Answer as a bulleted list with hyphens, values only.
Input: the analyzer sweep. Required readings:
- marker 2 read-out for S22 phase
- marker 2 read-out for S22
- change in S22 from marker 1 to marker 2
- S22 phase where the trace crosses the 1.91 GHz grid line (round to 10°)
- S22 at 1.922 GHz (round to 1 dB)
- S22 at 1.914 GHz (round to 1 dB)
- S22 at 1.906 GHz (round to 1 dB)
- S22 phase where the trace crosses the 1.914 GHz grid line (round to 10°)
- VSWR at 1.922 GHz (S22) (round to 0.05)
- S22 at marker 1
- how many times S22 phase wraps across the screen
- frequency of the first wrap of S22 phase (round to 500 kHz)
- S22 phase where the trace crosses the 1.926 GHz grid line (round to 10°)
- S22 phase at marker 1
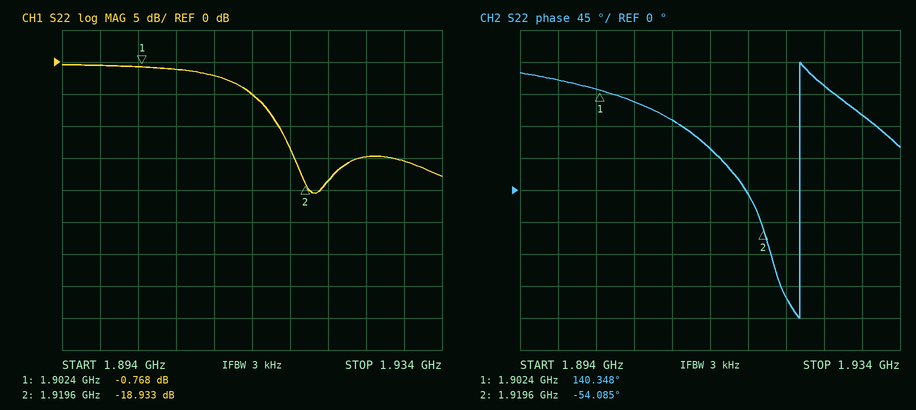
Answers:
- -54.085°
- -18.933 dB
- -18.165 dB
- 100°
- -19 dB
- -5 dB
- -1 dB
- 60°
- 1.25
- -0.768 dB
- 1
- 1.9235 GHz
- 150°
- 140.348°
